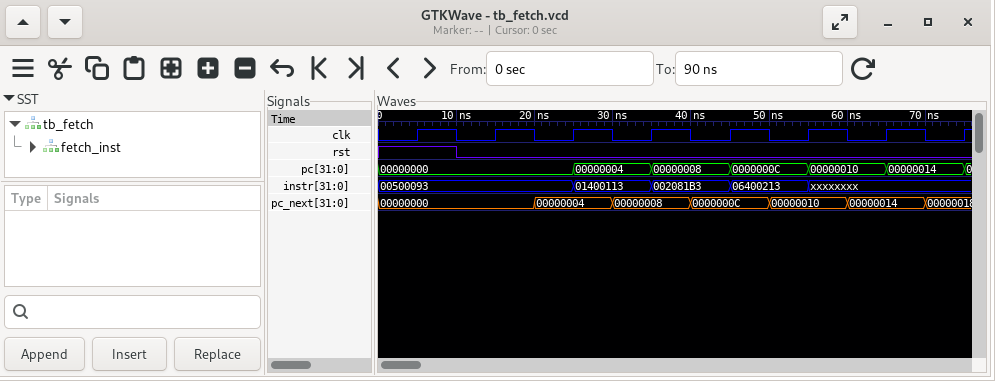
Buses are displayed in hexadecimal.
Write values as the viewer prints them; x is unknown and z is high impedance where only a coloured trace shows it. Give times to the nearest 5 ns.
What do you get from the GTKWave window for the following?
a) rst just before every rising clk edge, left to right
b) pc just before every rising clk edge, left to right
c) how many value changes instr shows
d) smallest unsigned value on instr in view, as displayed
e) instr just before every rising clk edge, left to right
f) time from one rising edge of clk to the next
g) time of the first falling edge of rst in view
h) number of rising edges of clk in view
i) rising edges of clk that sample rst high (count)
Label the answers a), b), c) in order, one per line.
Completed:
a) 1 0 0 0 0 0 0 0
b) 00000000, 00000000, 00000000, 00000004, 00000008, 0000000C, 00000010, 00000014
c) 4
d) 002081B3
e) 00500093, 00500093, 00500093, 01400113, 002081B3, 06400213, xxxxxxxx, xxxxxxxx
f) 10 ns
g) 10 ns
h) 8
i) 1
